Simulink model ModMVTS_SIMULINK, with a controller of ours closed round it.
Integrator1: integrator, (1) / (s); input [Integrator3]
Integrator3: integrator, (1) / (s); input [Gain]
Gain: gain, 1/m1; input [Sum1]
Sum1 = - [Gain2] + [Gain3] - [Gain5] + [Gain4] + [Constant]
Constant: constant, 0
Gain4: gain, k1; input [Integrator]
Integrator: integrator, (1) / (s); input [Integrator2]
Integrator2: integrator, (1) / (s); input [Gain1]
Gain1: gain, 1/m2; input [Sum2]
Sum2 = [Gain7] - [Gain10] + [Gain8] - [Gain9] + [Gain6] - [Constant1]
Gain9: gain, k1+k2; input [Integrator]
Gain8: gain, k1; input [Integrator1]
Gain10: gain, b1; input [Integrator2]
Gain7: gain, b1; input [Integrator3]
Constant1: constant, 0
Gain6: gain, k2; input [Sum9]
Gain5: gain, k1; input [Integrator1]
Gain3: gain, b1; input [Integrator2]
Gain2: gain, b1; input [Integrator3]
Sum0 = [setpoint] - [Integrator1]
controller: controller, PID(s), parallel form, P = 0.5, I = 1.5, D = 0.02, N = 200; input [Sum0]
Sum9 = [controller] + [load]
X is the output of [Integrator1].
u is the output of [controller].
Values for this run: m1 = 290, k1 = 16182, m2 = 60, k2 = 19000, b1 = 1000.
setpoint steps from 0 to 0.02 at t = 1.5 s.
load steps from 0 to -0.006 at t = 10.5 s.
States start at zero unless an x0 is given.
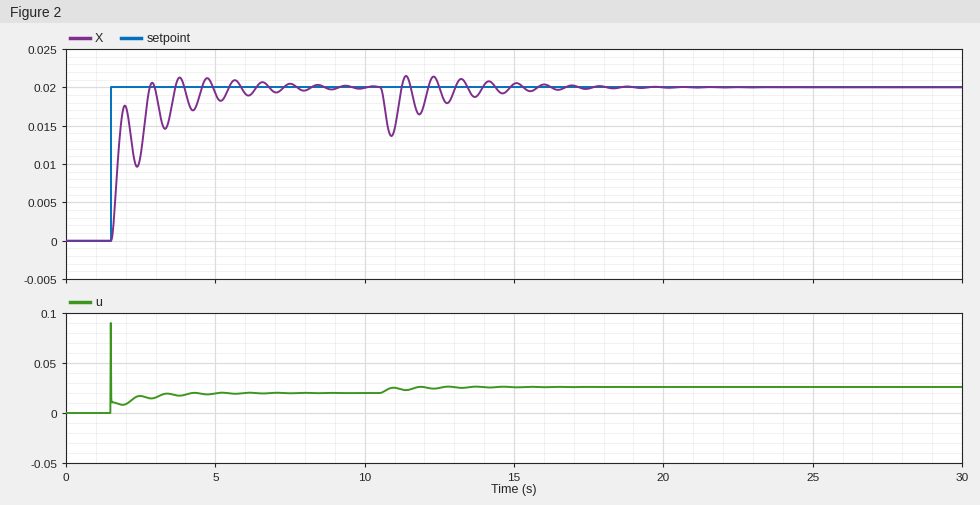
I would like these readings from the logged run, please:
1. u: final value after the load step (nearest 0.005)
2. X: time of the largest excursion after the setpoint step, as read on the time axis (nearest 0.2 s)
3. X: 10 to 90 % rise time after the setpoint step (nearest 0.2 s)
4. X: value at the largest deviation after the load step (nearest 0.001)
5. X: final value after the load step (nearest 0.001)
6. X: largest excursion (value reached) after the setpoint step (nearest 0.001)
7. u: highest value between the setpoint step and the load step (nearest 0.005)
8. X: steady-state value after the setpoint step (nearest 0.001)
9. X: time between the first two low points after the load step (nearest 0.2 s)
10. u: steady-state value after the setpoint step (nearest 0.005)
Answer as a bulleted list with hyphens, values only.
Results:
- 0.025
- 3.8 s
- 1.2 s
- 0.014
- 0.020
- 0.021
- 0.090
- 0.020
- 1.0 s
- 0.020
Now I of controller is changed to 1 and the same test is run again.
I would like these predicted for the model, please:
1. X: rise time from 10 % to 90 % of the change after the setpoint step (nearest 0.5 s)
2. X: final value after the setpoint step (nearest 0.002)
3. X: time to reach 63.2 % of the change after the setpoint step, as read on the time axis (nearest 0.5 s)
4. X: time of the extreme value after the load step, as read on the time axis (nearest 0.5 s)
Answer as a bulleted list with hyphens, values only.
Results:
- 2.0 s
- 0.020
- 2.0 s
- 11.0 s
